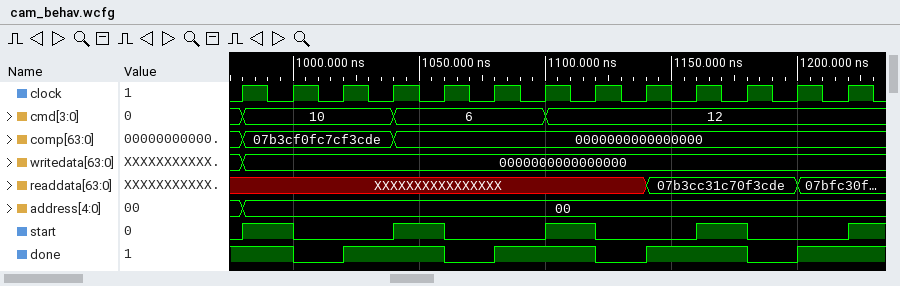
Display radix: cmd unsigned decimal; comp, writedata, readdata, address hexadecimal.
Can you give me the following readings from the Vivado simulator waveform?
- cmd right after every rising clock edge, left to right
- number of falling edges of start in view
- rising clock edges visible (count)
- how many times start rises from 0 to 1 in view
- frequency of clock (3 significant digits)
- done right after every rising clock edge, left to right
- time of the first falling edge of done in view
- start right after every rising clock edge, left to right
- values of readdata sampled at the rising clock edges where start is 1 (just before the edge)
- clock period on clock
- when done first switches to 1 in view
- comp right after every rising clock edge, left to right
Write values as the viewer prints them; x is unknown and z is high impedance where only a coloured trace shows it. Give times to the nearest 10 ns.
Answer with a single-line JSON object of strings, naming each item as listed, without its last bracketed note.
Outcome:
{"cmd right after every rising clock edge, left to right": "10, 10, 10, 6, 6, 6, 12, 12, 12, 12, 12, 12, 12", "number of falling edges of start in view": "4", "rising clock edges visible": "13", "how many times start rises from 0 to 1 in view": "5", "frequency of clock": "50.0 MHz", "done right after every rising clock edge, left to right": "1 0 1 1 0 1 1 0 1 1 0 1 1", "time of the first falling edge of done in view": "1000 ns", "start right after every rising clock edge, left to right": "1 0 0 1 0 0 1 0 0 1 0 0 1", "values of readdata sampled at the rising clock edges where start is 1": "XXXXXXXXXXXXXXXX, XXXXXXXXXXXXXXXX, XXXXXXXXXXXXXXXX, 07b3cc31c70f3cde", "clock period on clock": "20 ns", "when done first switches to 1 in view": "1020 ns", "comp right after every rising clock edge, left to right": "07b3cf0fc7cf3cde, 07b3cf0fc7cf3cde, 07b3cf0fc7cf3cde, 0000000000000000, 0000000000000000, 0000000000000000, 0000000000000000, 0000000000000000, 0000000000000000, 0000000000000000, 0000000000000000, 0000000000000000, 0000000000000000"}
